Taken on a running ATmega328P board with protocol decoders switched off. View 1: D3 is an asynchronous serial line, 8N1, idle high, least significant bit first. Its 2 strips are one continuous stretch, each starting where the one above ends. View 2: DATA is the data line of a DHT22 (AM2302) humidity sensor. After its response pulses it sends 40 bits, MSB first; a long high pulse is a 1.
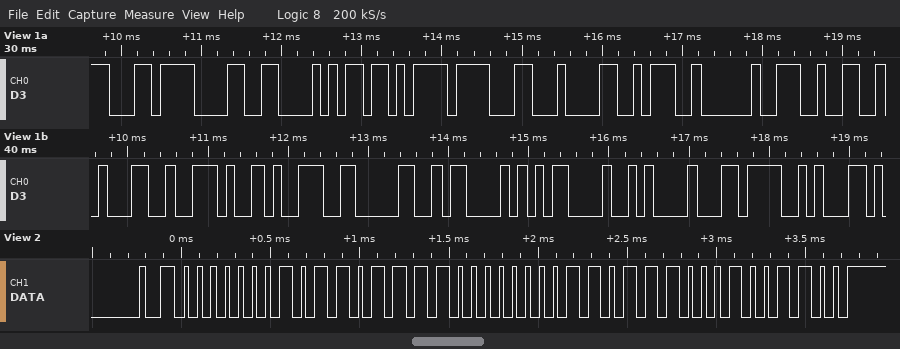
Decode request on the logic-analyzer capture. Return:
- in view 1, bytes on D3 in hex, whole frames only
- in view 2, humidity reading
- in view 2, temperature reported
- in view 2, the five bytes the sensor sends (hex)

EC 98 A8 EB 8F 84 3A 20 32 31 2E 39 30 43 0D 0A EC 8A
36.7 %
22.0 °C
01 6F 00 DC 4C
